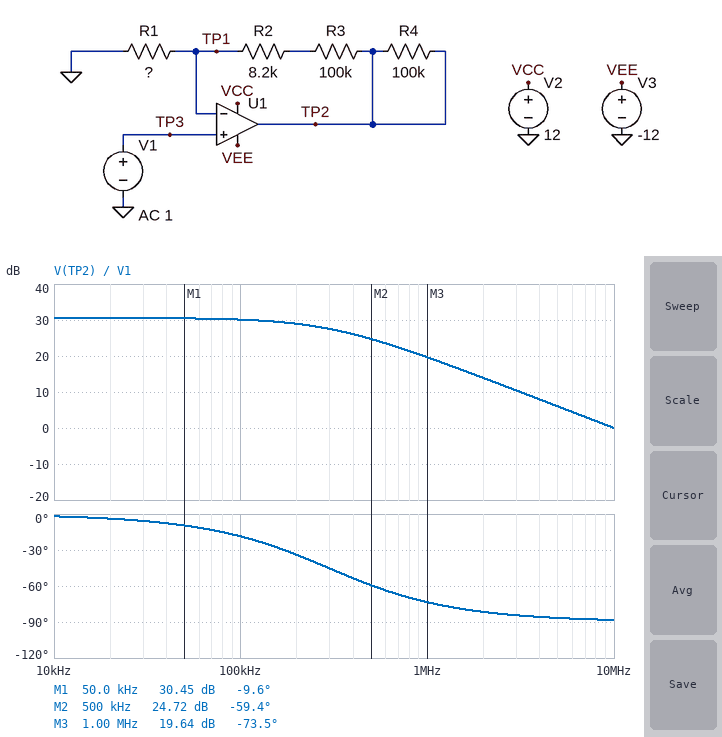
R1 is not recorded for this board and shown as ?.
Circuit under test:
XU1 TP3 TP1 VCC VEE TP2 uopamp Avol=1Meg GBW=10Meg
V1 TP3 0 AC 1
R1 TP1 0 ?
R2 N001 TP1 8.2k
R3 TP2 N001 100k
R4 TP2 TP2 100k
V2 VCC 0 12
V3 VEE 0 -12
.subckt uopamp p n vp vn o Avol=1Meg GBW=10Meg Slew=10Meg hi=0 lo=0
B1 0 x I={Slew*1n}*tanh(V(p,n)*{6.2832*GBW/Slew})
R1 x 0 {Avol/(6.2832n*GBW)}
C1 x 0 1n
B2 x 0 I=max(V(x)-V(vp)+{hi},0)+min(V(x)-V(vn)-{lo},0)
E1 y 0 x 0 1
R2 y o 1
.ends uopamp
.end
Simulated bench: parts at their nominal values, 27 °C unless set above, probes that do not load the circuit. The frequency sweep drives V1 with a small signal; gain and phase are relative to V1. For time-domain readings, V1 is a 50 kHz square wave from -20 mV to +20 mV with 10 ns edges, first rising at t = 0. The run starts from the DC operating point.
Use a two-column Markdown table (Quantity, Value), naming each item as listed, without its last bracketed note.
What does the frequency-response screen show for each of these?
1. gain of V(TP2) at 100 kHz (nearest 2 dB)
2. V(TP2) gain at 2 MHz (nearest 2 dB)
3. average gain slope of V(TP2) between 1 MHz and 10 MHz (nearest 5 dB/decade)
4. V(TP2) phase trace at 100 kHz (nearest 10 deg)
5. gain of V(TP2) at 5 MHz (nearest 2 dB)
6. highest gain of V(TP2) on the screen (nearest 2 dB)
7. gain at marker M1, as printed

| Quantity | Value |
|---|---|
| gain of V(TP2) at 100 kHz | 30 dB |
| V(TP2) gain at 2 MHz | 14 dB |
| average gain slope of V(TP2) between 1 MHz and 10 MHz | -20 dB/decade |
| V(TP2) phase trace at 100 kHz | -20 deg |
| gain of V(TP2) at 5 MHz | 6 dB |
| highest gain of V(TP2) on the screen | 30 dB |
| gain at marker M1, as printed | 30.45 dB |
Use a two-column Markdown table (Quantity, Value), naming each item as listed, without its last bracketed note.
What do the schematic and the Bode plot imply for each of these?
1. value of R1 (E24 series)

| Quantity | Value |
|---|---|
| value of R1 | 3.3 kΩ |
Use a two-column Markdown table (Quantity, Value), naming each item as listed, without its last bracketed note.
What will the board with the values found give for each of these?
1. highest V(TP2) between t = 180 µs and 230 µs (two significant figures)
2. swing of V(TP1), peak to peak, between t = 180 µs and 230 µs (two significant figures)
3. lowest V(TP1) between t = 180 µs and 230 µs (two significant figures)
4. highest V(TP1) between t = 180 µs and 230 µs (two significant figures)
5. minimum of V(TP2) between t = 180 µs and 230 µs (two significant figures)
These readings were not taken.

| Quantity | Value |
|---|---|
| highest V(TP2) between t = 180 µs and 230 µs | 680 mV |
| swing of V(TP1), peak to peak, between t = 180 µs and 230 µs | 40 mV |
| lowest V(TP1) between t = 180 µs and 230 µs | -20 mV |
| highest V(TP1) between t = 180 µs and 230 µs | 20 mV |
| minimum of V(TP2) between t = 180 µs and 230 µs | -680 mV |
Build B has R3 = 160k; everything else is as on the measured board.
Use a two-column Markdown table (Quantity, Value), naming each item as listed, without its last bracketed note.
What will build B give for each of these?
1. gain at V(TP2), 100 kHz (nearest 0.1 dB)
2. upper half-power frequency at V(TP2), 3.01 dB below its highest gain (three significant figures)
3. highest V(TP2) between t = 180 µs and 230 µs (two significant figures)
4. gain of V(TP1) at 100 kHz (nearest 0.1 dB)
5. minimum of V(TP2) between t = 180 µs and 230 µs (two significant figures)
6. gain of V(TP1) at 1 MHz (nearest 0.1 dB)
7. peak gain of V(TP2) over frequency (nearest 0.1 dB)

| Quantity | Value |
|---|---|
| gain at V(TP2), 100 kHz | 33.3 dB |
| upper half-power frequency at V(TP2), 3.01 dB below its highest gain | 192 kHz |
| highest V(TP2) between t = 180 µs and 230 µs | 1.0 V |
| gain of V(TP1) at 100 kHz | -1.0 dB |
| minimum of V(TP2) between t = 180 µs and 230 µs | -1.0 V |
| gain of V(TP1) at 1 MHz | -14.5 dB |
| peak gain of V(TP2) over frequency | 34.3 dB |
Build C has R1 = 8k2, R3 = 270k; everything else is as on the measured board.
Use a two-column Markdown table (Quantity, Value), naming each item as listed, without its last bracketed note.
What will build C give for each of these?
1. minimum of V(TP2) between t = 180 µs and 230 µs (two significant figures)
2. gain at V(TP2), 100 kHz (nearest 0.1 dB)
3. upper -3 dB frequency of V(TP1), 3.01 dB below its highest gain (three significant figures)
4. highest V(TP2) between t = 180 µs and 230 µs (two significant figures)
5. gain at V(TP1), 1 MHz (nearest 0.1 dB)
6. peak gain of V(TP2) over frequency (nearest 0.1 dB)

| Quantity | Value |
|---|---|
| minimum of V(TP2) between t = 180 µs and 230 µs | -700 mV |
| gain at V(TP2), 100 kHz | 30.4 dB |
| upper -3 dB frequency of V(TP1), 3.01 dB below its highest gain | 286 kHz |
| highest V(TP2) between t = 180 µs and 230 µs | 700 mV |
| gain at V(TP1), 1 MHz | -11.2 dB |
| peak gain of V(TP2) over frequency | 30.9 dB |
